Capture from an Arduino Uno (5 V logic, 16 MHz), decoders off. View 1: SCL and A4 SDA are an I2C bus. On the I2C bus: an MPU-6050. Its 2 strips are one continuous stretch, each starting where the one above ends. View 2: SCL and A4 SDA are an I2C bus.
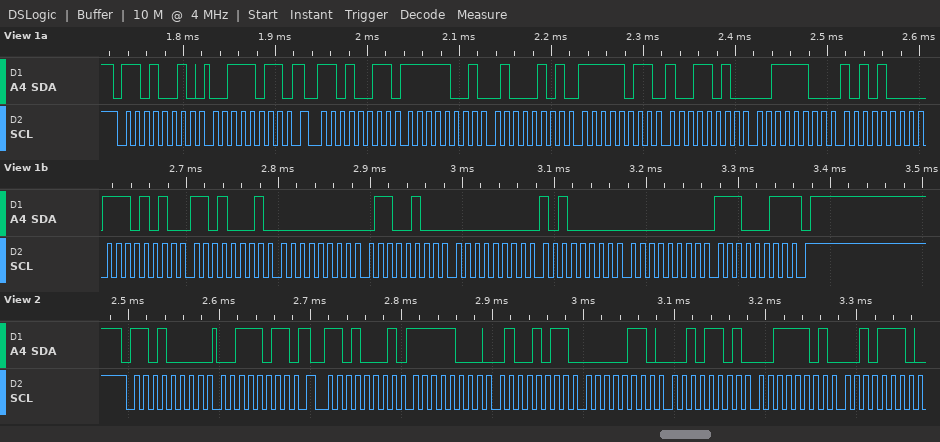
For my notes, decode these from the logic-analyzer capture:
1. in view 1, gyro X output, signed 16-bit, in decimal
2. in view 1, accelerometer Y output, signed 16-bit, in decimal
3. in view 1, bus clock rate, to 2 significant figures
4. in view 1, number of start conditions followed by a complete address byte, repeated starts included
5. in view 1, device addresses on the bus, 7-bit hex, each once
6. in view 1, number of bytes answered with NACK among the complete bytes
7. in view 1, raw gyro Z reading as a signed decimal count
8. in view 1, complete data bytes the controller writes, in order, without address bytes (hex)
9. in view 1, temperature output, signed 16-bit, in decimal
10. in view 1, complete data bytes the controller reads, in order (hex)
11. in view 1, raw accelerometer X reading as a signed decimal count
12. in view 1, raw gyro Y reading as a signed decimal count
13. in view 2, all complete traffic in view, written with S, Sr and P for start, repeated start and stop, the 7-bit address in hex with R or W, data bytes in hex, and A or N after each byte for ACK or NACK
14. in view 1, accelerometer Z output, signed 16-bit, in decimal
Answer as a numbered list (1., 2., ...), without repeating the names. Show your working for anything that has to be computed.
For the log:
1. 0x0064 = 100
2. 0xFB9A = -1126
3. 100 kHz
4. 2
5. 0x69
6. 1
7. 0x00E3 = 227
8. 3B
9. 0xEAD1 = -5423
10. F9 45 FB 9A 3C A8 EA D1 00 64 00 A0 00 E3
11. 0xF945 = -1723
12. 0x00A0 = 160
13. S 68W A 3B A Sr 68R A F8 A 4B A 06 A 2D A 3D A 2E A
14. 0x3CA8 = 15528
